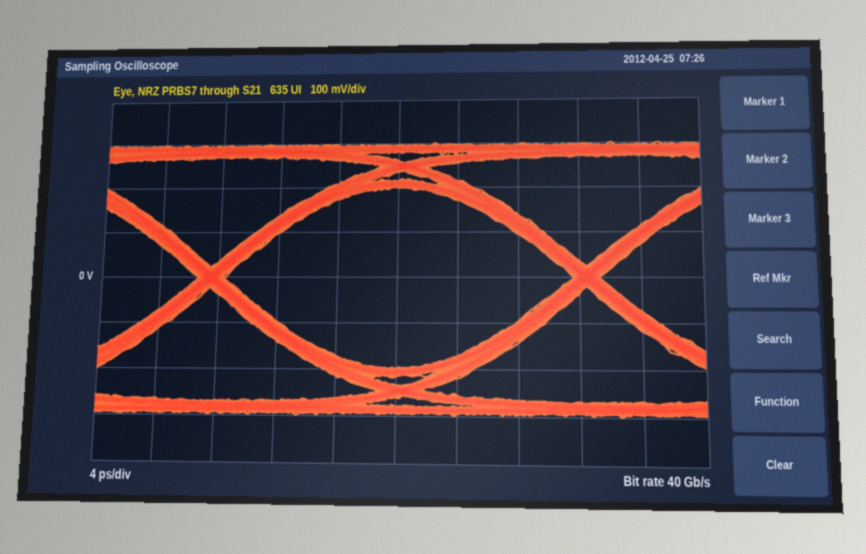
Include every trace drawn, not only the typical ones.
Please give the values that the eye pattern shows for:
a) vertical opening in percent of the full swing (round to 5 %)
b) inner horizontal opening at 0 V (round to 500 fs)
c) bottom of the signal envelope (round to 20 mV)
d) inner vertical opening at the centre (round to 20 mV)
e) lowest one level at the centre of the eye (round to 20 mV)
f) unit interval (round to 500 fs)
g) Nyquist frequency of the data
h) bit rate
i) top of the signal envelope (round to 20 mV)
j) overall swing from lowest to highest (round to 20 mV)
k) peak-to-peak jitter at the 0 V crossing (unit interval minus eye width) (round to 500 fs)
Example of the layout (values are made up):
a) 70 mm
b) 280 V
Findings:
a) 65 %
b) 23.0 ps
c) -300 mV
d) 400 mV
e) 200 mV
f) 25.0 ps
g) 20 GHz
h) 40 Gb/s
i) 300 mV
j) 600 mV
k) 2.0 ps
